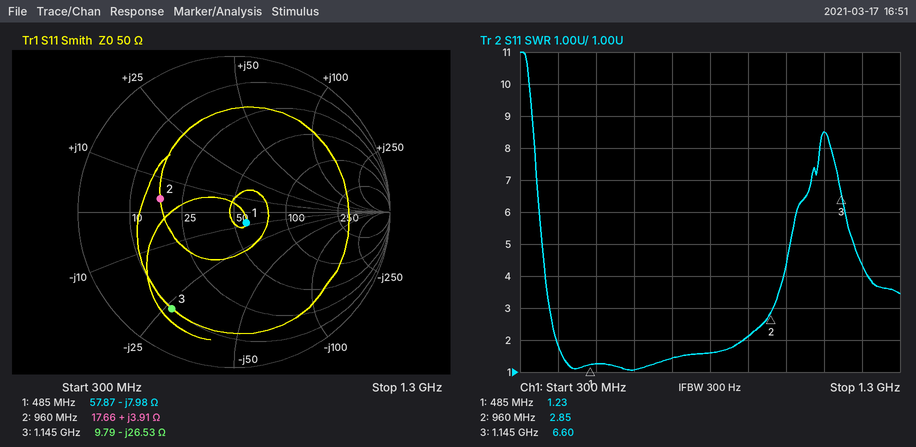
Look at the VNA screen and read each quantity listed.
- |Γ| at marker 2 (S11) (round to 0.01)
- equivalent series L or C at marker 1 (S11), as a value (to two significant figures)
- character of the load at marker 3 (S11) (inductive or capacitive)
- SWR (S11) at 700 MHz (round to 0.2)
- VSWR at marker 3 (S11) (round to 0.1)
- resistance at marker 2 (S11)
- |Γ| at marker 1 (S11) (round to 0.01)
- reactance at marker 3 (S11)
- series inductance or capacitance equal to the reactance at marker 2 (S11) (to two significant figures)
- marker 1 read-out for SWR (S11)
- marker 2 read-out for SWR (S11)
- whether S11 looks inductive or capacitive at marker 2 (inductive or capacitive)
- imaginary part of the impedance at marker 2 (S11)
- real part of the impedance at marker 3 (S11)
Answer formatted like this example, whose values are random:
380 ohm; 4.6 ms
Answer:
0.48; 41 pF; capacitive; 1.4; 6.6; 17.66 Ω; 0.10; -26.53 Ω; 650 pH; 1.23; 2.85; inductive; +3.91 Ω; 9.79 Ω
